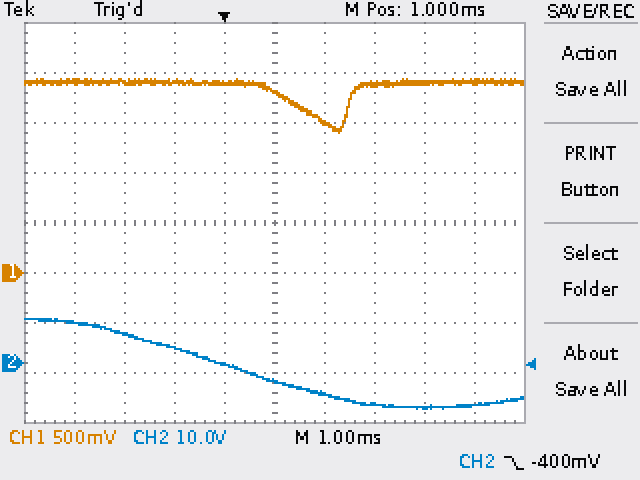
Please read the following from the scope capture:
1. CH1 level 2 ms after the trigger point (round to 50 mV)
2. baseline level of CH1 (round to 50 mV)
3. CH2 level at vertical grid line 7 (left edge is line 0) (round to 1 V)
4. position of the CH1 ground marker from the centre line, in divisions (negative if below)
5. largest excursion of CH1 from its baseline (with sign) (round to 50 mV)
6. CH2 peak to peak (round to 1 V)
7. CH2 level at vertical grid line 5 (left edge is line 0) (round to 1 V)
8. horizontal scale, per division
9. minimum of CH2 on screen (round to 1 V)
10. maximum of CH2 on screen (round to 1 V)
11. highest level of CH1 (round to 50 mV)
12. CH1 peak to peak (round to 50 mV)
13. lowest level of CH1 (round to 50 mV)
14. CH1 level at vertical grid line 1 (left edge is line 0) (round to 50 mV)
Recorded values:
1.50 V
1.90 V
-8 V
-1.0 div
-500 mV
18 V
-4 V
1 ms
-9 V
9 V
1.95 V
550 mV
1.40 V
1.90 V
